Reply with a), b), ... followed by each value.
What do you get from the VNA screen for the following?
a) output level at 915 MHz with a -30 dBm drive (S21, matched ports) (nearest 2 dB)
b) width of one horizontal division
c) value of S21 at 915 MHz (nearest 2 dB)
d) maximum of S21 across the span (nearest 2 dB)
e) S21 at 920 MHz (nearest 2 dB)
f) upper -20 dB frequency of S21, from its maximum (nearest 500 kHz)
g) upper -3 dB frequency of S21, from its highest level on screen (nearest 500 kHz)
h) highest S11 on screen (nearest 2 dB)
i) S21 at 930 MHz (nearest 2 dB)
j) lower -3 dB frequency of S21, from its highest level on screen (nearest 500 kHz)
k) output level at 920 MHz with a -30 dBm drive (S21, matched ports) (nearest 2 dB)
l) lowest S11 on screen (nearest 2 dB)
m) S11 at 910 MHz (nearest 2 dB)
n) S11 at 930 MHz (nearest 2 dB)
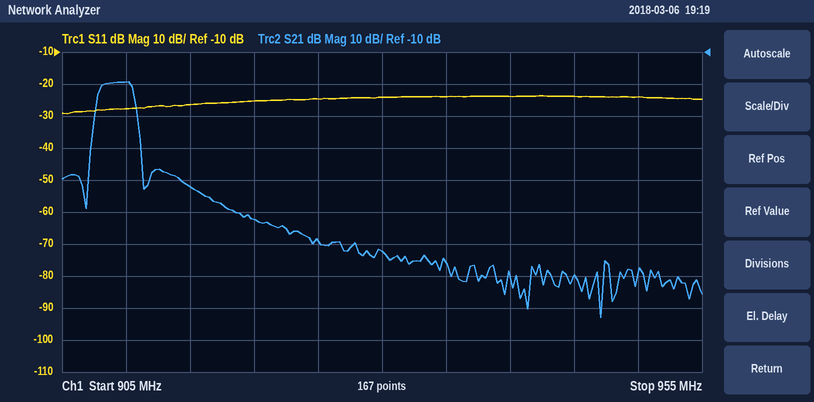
a) -82 dBm
b) 5 MHz
c) -52 dB
d) -20 dB
e) -62 dB
f) 911.0 MHz
g) 910.5 MHz
h) -24 dB
i) -72 dB
j) 908.0 MHz
k) -92 dBm
l) -30 dB
m) -28 dB
n) -24 dB
